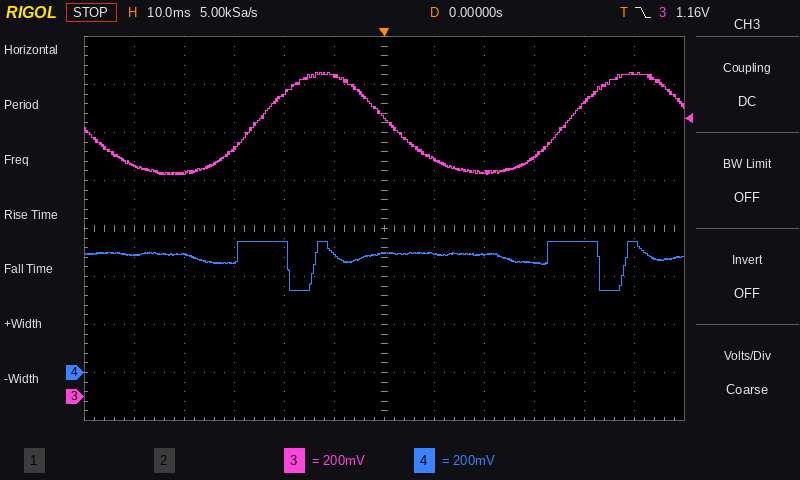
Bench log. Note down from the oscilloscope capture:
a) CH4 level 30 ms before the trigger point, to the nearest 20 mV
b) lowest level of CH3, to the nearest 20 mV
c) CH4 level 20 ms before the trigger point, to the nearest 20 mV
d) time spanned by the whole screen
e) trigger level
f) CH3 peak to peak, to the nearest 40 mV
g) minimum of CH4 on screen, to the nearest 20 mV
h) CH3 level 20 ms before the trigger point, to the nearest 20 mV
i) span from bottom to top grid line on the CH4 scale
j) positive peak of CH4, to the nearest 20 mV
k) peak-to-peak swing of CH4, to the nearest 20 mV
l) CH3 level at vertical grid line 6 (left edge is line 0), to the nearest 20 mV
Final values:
460 mV
920 mV
540 mV
120 ms
1.16 V
440 mV
340 mV
1.26 V
1.6 V
540 mV
200 mV
1.16 V
